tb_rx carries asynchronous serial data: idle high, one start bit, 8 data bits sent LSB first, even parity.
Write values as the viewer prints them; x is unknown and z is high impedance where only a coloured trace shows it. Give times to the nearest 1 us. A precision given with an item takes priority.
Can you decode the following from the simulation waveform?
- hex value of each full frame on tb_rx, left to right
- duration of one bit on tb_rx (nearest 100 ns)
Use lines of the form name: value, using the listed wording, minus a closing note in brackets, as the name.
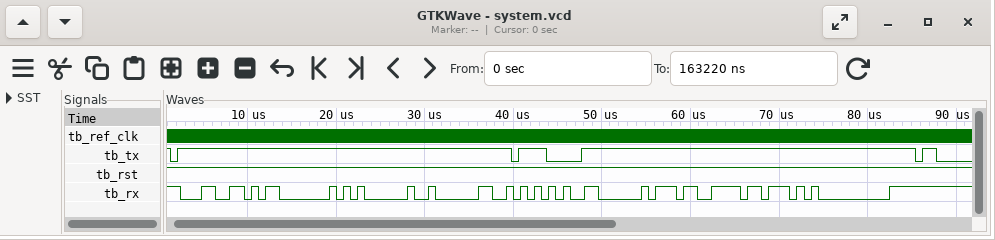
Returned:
hex value of each full frame on tb_rx, left to right: CC, 03, 05, 02, AA, 06, 37, BB, 00
duration of one bit on tb_rx: 800 ns
